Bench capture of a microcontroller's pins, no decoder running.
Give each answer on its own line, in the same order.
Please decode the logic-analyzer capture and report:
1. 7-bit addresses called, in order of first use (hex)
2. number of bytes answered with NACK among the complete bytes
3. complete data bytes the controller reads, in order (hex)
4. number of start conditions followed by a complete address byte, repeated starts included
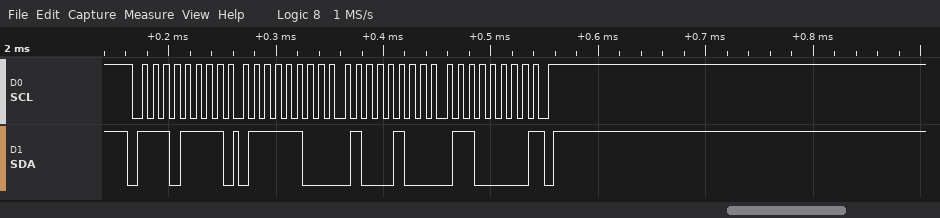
0x77
1
7C 44 60
1
